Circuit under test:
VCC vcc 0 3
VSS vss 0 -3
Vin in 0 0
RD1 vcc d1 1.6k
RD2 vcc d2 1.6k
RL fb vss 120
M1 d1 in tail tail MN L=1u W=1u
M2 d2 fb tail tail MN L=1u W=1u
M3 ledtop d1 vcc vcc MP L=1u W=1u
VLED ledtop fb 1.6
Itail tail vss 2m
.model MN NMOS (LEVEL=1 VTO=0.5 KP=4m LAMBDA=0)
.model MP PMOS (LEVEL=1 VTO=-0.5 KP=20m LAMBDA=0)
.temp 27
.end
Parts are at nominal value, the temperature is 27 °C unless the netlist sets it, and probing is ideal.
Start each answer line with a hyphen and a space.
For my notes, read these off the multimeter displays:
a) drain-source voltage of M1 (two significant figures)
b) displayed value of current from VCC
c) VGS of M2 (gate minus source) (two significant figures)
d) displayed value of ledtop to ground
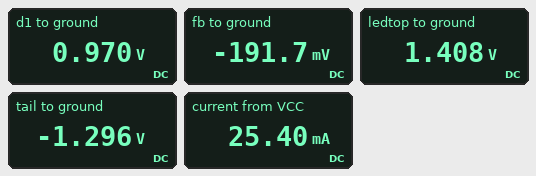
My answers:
- 2.3 V
- 25.40 mA
- 1.1 V
- 1.408 V
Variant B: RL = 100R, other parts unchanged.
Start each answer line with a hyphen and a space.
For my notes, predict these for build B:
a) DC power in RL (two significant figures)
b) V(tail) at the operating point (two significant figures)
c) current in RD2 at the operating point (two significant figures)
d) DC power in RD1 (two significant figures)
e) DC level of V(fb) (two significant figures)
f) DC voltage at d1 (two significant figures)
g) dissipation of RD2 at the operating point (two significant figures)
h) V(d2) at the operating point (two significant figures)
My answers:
- 76 mW
- -1.3 V
- 650 µA
- 2.9 mW
- -250 mV
- 840 mV
- 680 µW
- 2.0 V
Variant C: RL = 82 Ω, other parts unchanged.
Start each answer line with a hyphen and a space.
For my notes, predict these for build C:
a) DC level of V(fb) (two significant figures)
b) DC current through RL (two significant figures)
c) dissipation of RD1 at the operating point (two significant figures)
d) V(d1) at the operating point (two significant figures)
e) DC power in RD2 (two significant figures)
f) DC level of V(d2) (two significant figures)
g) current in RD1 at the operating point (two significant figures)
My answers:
- -320 mV
- 33 mA
- 3.3 mW
- 690 mV
- 500 µW
- 2.1 V
- 1.4 mA
